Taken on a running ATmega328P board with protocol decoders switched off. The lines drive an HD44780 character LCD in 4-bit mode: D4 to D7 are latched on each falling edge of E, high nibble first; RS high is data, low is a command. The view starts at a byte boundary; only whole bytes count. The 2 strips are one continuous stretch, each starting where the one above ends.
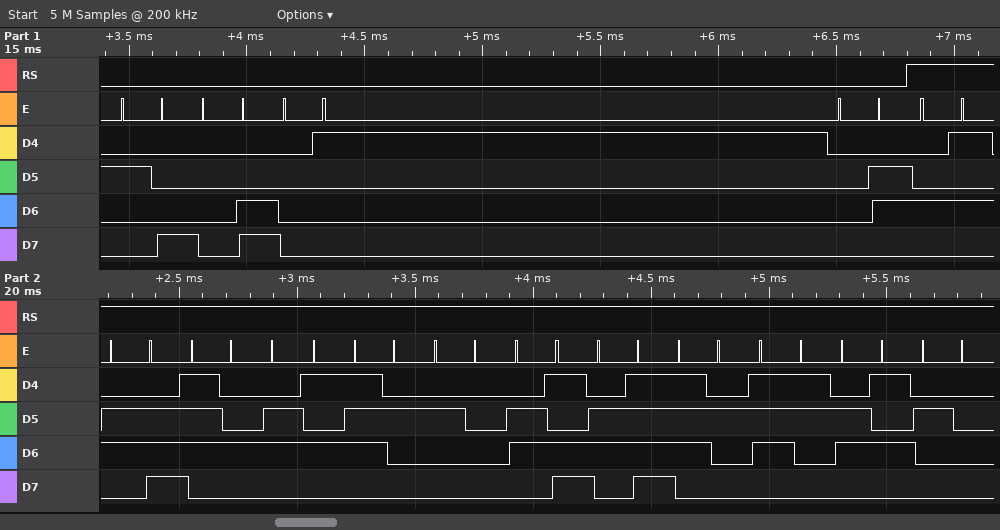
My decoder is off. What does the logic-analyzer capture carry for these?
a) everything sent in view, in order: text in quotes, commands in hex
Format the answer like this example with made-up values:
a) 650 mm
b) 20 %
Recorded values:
a) 0x28 0x0C 0x01 0x06 "Enter morse "
